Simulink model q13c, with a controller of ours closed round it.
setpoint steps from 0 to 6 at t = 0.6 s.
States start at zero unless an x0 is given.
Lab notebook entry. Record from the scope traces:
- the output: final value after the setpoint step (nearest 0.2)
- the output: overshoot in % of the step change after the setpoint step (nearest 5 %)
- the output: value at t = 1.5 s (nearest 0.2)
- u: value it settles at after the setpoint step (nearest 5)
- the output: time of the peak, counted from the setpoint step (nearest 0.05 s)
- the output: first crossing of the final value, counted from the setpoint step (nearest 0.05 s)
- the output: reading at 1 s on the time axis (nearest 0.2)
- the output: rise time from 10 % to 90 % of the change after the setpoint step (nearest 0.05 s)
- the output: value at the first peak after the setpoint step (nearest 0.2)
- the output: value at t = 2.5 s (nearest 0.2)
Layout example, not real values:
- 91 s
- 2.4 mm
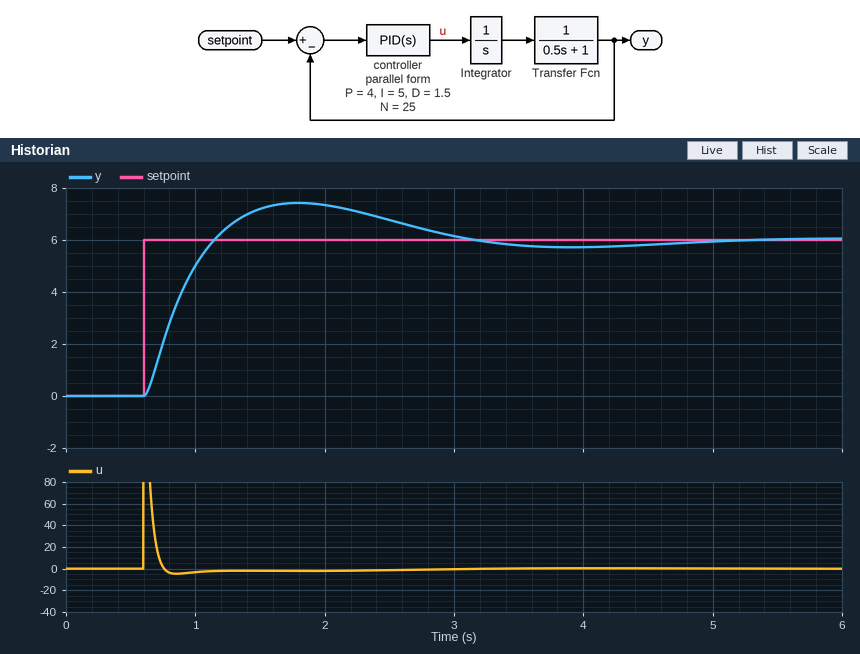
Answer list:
- 6.0
- 25 %
- 7.2
- 0
- 1.20 s
- 0.55 s
- 5.0
- 0.40 s
- 7.4
- 6.8
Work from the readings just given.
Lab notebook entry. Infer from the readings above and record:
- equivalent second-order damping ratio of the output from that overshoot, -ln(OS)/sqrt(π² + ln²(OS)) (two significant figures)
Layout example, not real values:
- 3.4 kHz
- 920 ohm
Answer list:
- 0.40
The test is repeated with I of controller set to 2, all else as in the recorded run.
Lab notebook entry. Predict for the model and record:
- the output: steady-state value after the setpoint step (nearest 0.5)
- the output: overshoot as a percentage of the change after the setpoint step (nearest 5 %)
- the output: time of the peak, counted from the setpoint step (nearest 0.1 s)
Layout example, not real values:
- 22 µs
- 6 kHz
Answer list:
- 6.0
- 10 %
- 1.3 s
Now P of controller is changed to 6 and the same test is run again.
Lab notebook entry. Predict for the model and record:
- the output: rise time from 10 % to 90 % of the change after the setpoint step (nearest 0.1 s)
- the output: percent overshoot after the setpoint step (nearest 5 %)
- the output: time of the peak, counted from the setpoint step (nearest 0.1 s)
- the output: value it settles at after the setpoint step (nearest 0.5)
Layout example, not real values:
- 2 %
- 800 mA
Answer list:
- 0.3 s
- 20 %
- 0.9 s
- 6.0
